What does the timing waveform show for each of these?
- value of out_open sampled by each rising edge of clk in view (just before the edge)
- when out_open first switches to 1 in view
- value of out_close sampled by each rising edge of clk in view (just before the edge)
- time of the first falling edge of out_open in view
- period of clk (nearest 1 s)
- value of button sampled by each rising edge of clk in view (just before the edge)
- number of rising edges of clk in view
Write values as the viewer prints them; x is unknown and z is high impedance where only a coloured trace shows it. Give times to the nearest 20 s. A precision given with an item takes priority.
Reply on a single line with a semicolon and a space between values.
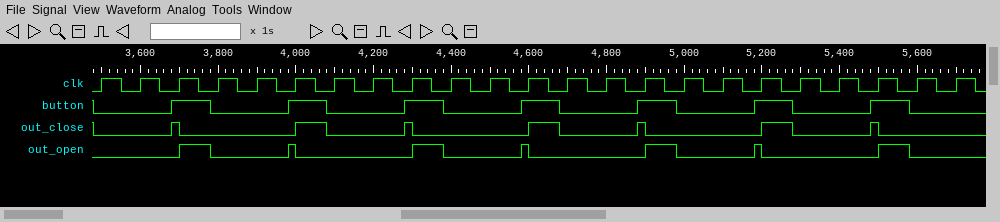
0 0 0 0 0 1 0 0 0 0 0 1 0 0 0 0 0 1 0 0 0 0 0; 3700 s; 0 0 1 0 0 0 0 0 1 0 0 0 0 0 1 0 0 0 0 0 1 0 0; 3780 s; 100 s; 0 0 1 0 0 1 0 0 1 0 0 1 0 0 1 0 0 1 0 0 1 0 0; 23
